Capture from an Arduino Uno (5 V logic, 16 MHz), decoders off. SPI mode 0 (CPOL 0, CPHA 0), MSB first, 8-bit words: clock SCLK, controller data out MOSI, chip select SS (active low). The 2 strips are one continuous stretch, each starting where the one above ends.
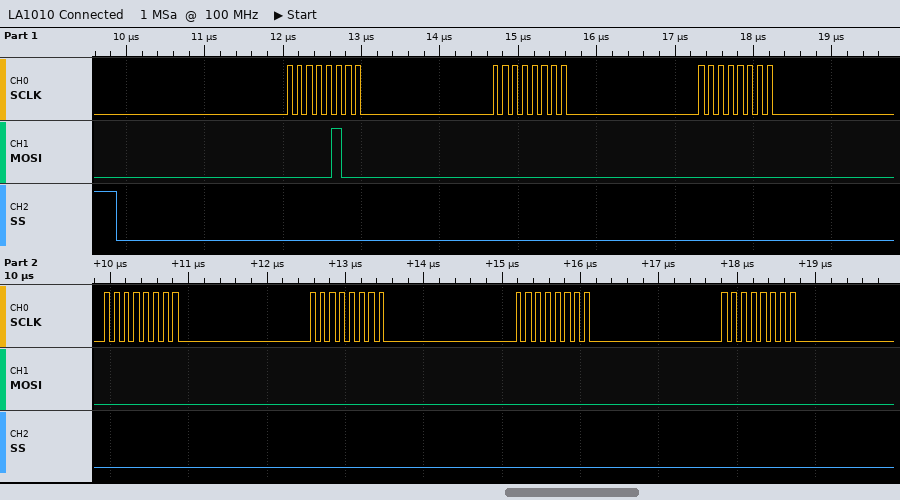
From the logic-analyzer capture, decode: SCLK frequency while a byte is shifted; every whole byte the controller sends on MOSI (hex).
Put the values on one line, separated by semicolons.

8 MHz; 0x04 0x00 0x00 0x00 0x00 0x00 0x00
